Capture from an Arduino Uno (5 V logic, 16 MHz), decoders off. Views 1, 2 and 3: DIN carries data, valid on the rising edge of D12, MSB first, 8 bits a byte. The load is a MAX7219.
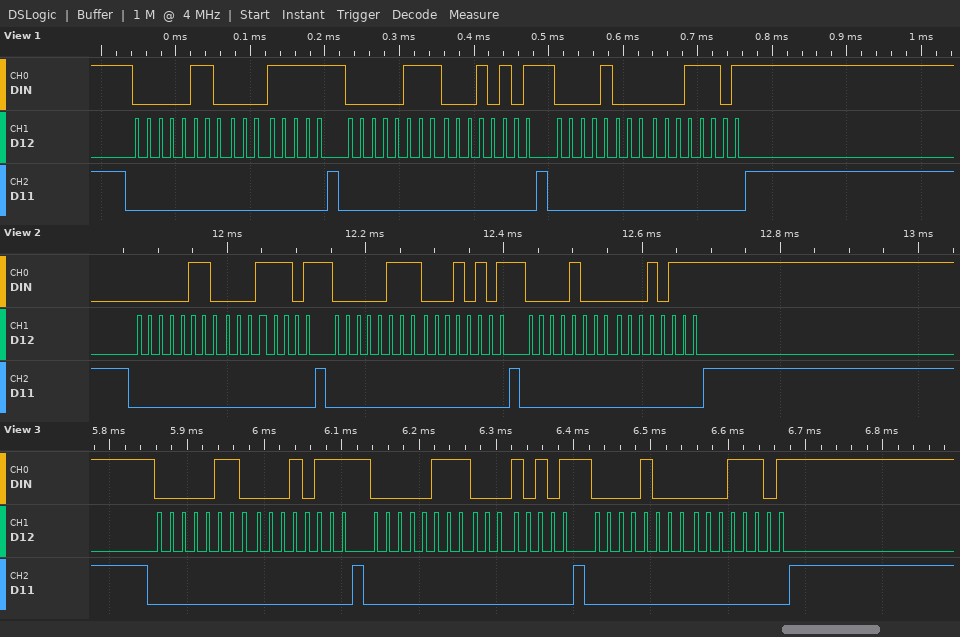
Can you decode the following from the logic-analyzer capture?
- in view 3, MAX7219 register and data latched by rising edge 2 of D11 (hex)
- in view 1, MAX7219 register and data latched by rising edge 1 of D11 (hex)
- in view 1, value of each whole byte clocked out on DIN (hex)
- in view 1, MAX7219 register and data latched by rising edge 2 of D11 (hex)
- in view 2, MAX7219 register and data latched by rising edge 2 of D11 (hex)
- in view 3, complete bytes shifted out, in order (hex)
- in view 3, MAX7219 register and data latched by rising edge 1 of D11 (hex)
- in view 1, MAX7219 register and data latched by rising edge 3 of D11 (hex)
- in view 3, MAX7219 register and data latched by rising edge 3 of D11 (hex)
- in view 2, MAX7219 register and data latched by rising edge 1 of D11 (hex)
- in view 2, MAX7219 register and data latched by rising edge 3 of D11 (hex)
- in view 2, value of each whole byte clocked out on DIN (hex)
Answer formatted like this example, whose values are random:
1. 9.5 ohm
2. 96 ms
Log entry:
1. register 0x7, data 0x15
2. register 0x6, data 0x1F
3. 0x06 0x1F 0x07 0x15 0x08 0x1D
4. register 0x7, data 0x15
5. register 0x7, data 0x15
6. 06 17 07 15 08 1D
7. register 0x6, data 0x17
8. register 0x8, data 0x1D
9. register 0x8, data 0x1D
10. register 0x6, data 0x1D
11. register 0x8, data 0x17
12. 06 1D 07 15 08 17
